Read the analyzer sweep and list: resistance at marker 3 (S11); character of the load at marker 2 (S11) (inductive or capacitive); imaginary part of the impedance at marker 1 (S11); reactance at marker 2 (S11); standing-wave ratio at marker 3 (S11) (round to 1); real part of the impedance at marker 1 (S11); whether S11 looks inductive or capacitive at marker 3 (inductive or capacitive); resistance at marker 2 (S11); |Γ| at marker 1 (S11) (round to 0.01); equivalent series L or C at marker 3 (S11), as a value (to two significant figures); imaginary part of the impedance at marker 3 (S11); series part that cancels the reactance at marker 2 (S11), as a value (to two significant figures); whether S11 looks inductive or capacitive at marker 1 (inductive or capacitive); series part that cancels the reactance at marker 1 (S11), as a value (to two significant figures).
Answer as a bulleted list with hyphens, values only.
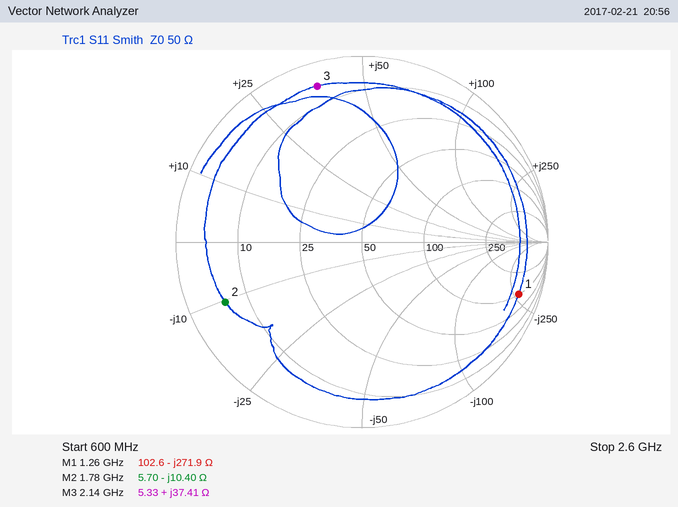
- 5.33 Ω
- capacitive
- -271.9 Ω
- -10.40 Ω
- 15
- 102.6 Ω
- inductive
- 5.70 Ω
- 0.89
- 2.8 nH
- +37.41 Ω
- 930 pH
- capacitive
- 34 nH
